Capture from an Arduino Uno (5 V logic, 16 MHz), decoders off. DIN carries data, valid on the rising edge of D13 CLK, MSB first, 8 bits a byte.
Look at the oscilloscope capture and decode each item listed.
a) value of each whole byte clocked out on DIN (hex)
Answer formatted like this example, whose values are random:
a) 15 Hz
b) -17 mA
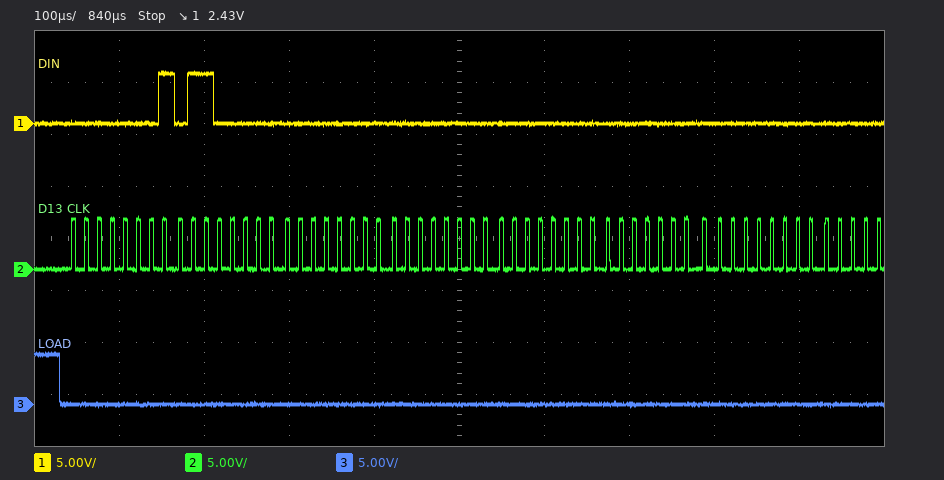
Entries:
a) 0x01 0x60 0x00 0x00 0x00 0x00 0x00
